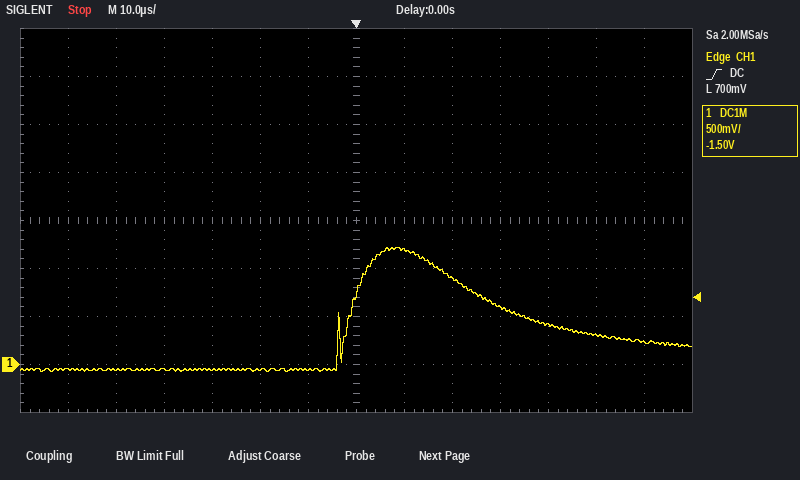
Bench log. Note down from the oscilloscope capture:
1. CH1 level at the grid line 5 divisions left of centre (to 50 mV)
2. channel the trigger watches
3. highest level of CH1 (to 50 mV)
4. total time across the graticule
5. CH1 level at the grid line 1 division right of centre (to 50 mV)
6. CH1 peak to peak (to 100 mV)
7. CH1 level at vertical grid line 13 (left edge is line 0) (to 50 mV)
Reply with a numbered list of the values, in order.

1. -50 mV
2. CH1
3. 1.20 V
4. 140 µs
5. 1.20 V
6. 1.30 V
7. 250 mV
